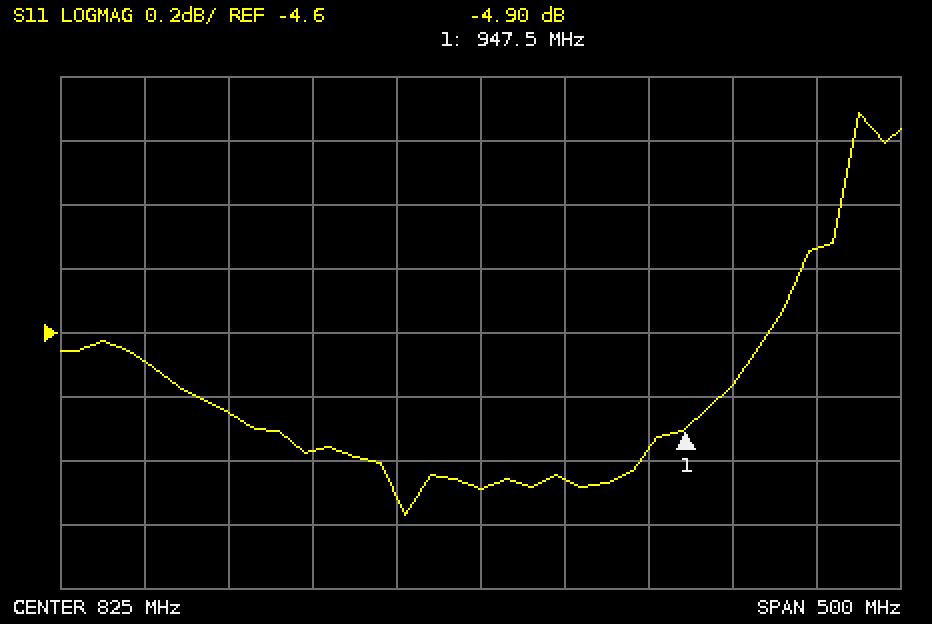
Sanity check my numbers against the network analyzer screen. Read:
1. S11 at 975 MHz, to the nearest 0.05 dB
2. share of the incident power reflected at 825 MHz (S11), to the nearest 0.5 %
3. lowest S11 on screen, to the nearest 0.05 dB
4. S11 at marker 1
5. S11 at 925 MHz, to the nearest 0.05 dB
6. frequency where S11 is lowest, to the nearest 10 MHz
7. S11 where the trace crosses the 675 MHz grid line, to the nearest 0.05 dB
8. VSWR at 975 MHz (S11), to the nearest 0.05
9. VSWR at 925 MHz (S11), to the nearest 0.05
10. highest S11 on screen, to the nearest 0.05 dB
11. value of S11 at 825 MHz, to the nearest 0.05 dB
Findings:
-4.75 dB
31.0 %
-5.15 dB
-4.90 dB
-4.95 dB
780 MHz
-4.85 dB
3.75
3.60
-3.90 dB
-5.10 dB
